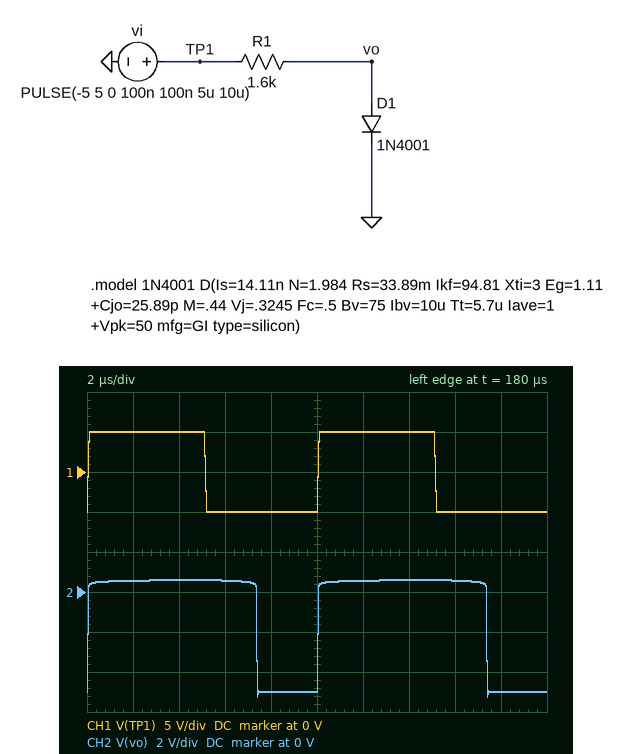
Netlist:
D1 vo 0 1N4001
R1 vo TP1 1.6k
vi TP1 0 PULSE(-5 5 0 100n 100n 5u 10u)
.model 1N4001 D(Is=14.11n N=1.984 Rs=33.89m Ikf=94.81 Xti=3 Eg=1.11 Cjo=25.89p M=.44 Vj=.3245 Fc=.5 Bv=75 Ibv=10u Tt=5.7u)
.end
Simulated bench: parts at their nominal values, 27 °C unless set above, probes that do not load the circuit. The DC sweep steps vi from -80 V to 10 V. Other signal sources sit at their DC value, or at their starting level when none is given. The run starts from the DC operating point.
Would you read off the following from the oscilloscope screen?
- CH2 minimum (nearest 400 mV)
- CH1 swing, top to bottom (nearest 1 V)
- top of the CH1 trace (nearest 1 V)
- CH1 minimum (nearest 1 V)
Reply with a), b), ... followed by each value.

a) -5.2 V
b) 10 V
c) 5 V
d) -5 V
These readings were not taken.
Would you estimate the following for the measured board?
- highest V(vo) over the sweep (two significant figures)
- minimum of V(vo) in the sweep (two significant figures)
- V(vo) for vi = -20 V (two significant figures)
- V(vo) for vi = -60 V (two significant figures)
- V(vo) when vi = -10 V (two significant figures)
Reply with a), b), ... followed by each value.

a) 660 mV
b) -76 V
c) -20 V
d) -60 V
e) -10 V
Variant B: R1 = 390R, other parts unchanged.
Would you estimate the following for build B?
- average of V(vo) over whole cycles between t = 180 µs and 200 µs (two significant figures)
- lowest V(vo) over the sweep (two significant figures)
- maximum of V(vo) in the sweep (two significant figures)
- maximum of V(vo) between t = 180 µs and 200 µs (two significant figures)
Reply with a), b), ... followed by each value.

a) -910 mV
b) -76 V
c) 740 mV
d) 670 mV
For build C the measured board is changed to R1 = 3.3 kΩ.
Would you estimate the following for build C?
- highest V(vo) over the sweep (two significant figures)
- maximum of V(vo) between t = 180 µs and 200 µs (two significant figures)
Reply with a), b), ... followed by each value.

a) 630 mV
b) 560 mV
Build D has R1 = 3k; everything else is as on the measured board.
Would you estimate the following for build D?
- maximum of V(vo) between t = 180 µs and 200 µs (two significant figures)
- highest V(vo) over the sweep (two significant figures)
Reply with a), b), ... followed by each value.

a) 570 mV
b) 630 mV
